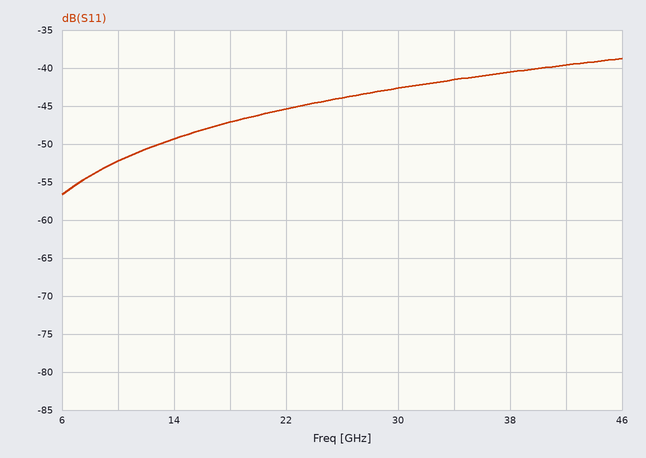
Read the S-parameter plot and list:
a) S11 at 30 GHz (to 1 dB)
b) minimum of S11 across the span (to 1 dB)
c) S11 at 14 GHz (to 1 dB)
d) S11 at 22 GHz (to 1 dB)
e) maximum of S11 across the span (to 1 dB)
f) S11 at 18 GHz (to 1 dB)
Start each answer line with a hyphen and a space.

- -43 dB
- -57 dB
- -49 dB
- -45 dB
- -39 dB
- -47 dB
